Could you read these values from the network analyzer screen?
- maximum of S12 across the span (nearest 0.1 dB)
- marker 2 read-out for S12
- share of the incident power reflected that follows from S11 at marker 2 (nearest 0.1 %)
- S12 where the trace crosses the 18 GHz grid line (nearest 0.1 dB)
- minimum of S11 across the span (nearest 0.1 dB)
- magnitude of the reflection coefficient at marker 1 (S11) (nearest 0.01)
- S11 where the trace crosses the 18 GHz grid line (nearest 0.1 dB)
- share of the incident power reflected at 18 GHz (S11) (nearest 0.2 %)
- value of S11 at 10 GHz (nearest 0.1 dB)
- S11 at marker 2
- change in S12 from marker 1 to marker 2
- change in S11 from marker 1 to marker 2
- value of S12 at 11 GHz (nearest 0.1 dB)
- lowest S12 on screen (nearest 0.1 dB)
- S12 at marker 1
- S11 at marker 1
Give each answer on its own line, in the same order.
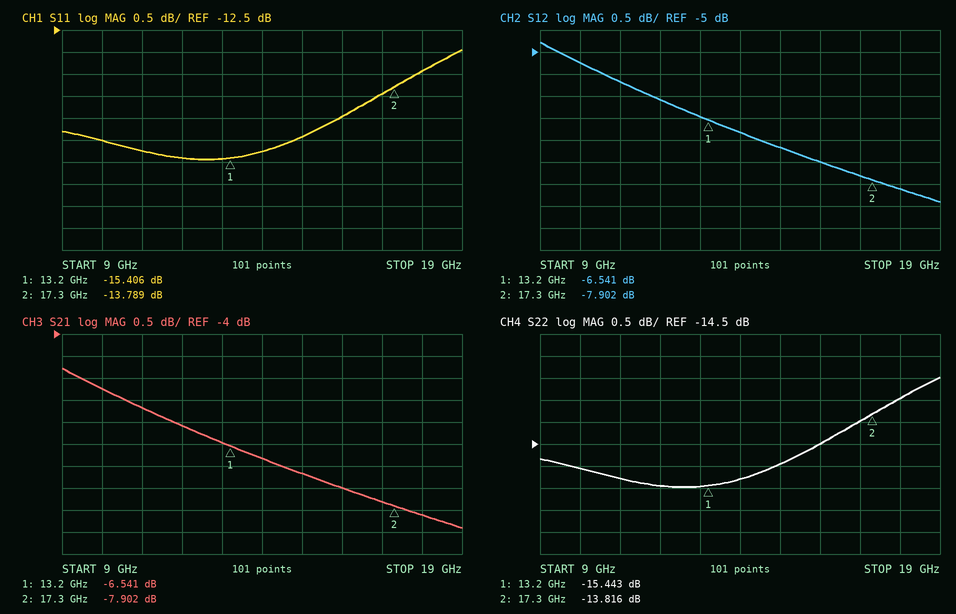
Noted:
-4.8 dB
-7.902 dB
4.2 %
-8.1 dB
-15.4 dB
0.17
-13.4 dB
4.6 %
-15.0 dB
-13.789 dB
-1.361 dB
1.617 dB
-5.7 dB
-8.4 dB
-6.541 dB
-15.406 dB
